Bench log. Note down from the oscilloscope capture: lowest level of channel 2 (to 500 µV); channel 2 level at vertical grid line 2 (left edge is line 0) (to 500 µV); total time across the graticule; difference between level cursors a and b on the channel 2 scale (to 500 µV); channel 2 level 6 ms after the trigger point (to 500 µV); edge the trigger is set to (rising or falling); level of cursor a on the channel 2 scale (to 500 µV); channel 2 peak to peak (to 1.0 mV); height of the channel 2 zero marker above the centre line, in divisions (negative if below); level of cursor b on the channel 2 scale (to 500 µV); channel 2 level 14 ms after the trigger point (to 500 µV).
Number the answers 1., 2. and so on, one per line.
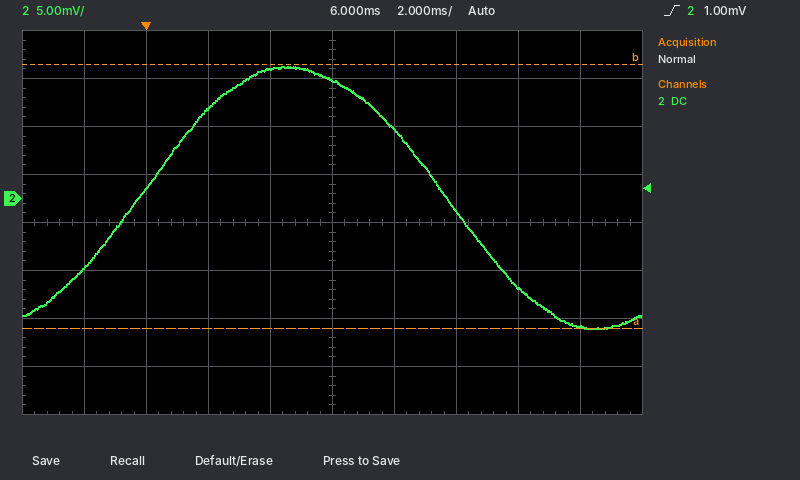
1. -13.5 mV
2. 1.0 mV
3. 20 ms
4. 27.5 mV
5. 12.5 mV
6. rising
7. -13.5 mV
8. 27.0 mV
9. +0.5 div
10. 14.0 mV
11. -13.5 mV
